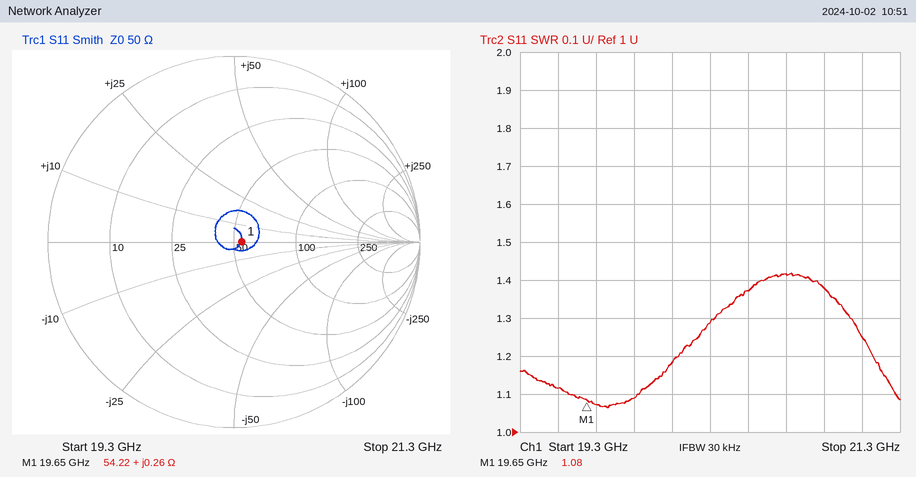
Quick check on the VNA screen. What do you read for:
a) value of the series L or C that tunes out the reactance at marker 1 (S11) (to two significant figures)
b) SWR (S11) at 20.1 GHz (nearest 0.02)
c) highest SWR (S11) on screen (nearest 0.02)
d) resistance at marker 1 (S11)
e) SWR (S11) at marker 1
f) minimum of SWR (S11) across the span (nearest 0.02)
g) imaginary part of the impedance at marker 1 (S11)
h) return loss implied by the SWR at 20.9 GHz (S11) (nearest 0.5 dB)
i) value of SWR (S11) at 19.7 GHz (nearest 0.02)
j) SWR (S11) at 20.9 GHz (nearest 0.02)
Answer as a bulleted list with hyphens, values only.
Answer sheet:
- 31 pF
- 1.18
- 1.42
- 54.22 Ω
- 1.08
- 1.06
- +0.26 Ω
- 16.0 dB
- 1.08
- 1.38
